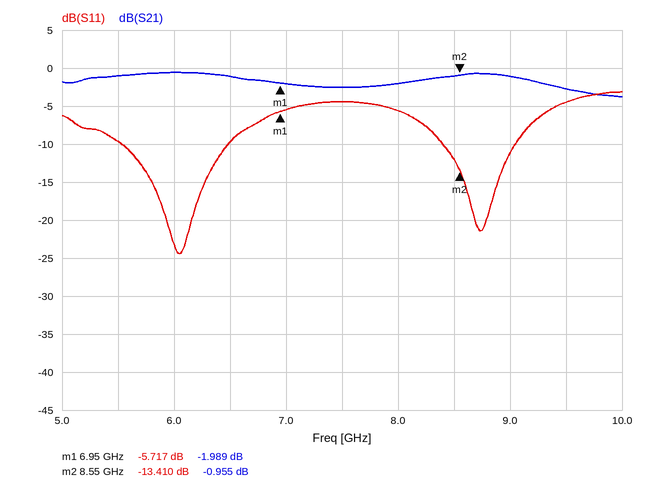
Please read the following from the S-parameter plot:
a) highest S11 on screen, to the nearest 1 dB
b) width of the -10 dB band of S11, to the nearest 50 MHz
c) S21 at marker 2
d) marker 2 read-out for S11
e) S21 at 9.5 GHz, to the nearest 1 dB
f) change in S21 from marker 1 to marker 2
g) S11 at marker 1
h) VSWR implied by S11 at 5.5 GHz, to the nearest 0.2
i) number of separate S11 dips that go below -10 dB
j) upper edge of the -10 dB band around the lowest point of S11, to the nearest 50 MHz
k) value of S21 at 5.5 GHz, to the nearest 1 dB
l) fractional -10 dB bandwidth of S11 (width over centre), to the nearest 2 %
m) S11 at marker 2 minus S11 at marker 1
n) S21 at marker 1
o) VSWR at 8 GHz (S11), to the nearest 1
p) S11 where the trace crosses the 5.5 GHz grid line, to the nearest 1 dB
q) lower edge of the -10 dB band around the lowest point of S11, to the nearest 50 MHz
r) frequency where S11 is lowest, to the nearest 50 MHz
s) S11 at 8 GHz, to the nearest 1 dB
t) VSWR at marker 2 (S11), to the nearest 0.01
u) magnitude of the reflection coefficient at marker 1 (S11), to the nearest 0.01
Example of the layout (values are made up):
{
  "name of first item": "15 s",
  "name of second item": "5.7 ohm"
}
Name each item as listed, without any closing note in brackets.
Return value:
{
  "highest S11 on screen, to the nearest 1 dB": "-3 dB",
  "width of the -10 dB band of S11, to the nearest 50 MHz": "950 MHz",
  "S21 at marker 2": "-0.955 dB",
  "marker 2 read-out for S11": "-13.410 dB",
  "S21 at 9.5 GHz, to the nearest 1 dB": "-3 dB",
  "change in S21 from marker 1 to marker 2": "1.034 dB",
  "S11 at marker 1": "-5.717 dB",
  "VSWR implied by S11 at 5.5 GHz, to the nearest 0.2": "2.0",
  "number of separate S11 dips that go below -10 dB": "2",
  "upper edge of the -10 dB band around the lowest point of S11, to the nearest 50 MHz": "6.50 GHz",
  "value of S21 at 5.5 GHz, to the nearest 1 dB": "-1 dB",
  "fractional -10 dB bandwidth of S11 (width over centre), to the nearest 2 %": "16 %",
  "S11 at marker 2 minus S11 at marker 1": "-7.693 dB",
  "S21 at marker 1": "-1.989 dB",
  "VSWR at 8 GHz (S11), to the nearest 1": "3",
  "S11 where the trace crosses the 5.5 GHz grid line, to the nearest 1 dB": "-10 dB",
  "lower edge of the -10 dB band around the lowest point of S11, to the nearest 50 MHz": "5.55 GHz",
  "frequency where S11 is lowest, to the nearest 50 MHz": "6.05 GHz",
  "S11 at 8 GHz, to the nearest 1 dB": "-6 dB",
  "VSWR at marker 2 (S11), to the nearest 0.01": "1.54",
  "magnitude of the reflection coefficient at marker 1 (S11), to the nearest 0.01": "0.52"
}
